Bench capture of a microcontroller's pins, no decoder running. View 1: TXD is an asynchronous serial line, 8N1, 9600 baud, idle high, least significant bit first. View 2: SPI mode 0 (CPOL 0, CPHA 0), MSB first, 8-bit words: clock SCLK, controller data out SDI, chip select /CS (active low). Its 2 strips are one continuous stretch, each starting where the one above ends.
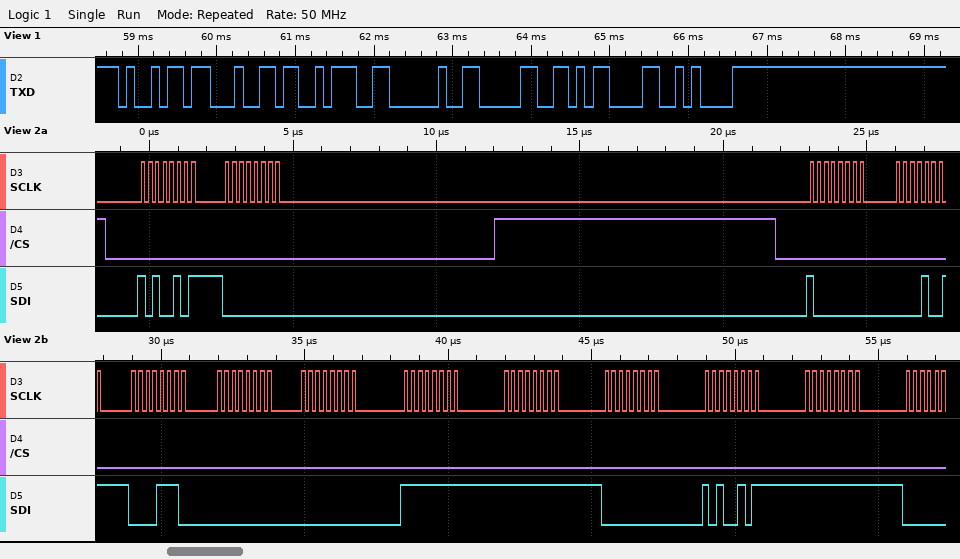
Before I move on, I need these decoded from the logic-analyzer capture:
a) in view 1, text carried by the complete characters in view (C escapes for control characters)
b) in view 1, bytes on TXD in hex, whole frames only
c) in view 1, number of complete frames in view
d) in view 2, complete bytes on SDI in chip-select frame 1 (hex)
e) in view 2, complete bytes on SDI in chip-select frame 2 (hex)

"id: 0\r\n"
69 64 3A 20 30 0D 0A
7
A5 00
80 09 0E 00 00 FF FF 00 A5 FF
